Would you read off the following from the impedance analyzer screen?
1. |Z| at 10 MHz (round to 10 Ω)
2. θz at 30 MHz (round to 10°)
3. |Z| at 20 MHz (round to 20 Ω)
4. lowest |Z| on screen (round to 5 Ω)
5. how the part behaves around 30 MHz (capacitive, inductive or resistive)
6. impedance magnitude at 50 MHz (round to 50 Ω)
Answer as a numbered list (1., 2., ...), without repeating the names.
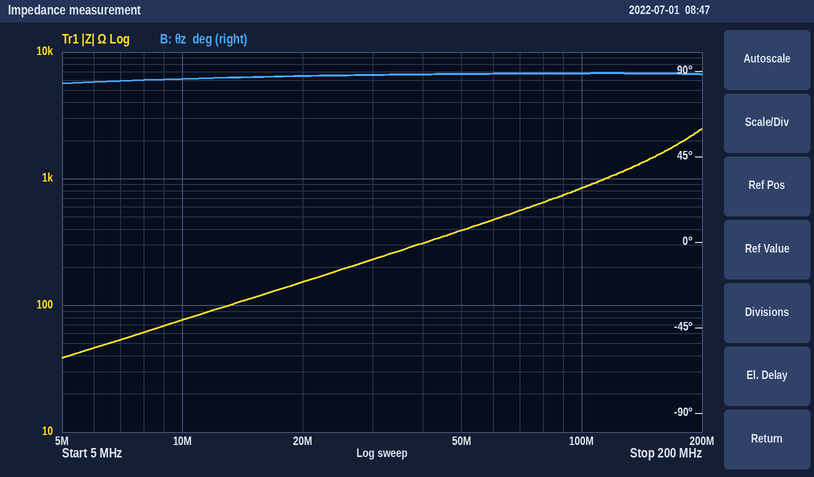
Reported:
1. 80 Ω
2. 90°
3. 160 Ω
4. 40 Ω
5. inductive
6. 400 Ω
